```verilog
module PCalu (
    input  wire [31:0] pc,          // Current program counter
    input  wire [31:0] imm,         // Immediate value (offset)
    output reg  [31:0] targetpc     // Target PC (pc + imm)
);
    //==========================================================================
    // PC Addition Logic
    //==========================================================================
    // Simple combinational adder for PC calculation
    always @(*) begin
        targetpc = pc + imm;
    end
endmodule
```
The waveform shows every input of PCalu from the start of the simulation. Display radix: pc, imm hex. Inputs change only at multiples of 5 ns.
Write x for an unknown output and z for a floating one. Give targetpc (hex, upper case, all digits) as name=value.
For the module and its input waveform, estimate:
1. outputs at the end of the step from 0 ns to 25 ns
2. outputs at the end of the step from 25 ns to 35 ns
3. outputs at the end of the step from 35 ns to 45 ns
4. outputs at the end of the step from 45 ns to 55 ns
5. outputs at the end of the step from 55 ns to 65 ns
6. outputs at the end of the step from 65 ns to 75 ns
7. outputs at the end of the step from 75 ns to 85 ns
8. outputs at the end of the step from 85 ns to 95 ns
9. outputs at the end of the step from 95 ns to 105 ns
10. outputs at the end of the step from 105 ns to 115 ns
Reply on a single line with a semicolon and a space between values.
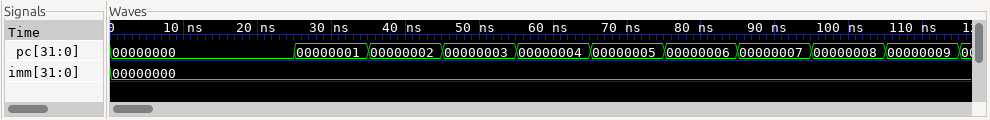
targetpc=00000000; targetpc=00000001; targetpc=00000002; targetpc=00000003; targetpc=00000004; targetpc=00000005; targetpc=00000006; targetpc=00000007; targetpc=00000008; targetpc=00000009
